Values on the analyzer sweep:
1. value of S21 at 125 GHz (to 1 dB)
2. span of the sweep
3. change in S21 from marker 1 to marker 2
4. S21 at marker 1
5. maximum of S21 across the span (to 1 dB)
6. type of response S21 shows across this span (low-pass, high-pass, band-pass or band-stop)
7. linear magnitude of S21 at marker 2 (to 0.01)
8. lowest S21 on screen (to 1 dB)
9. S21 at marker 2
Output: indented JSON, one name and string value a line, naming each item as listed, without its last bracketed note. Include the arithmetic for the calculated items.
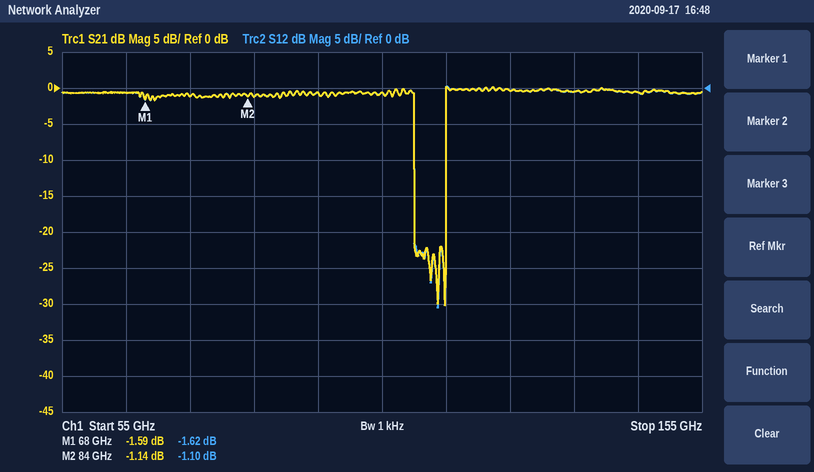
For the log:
{
  "value of S21 at 125 GHz": "0 dB",
  "span of the sweep": "100 GHz",
  "change in S21 from marker 1 to marker 2": "-1.14 − (-1.59) = 0.45 dB",
  "S21 at marker 1": "-1.59 dB",
  "maximum of S21 across the span": "0 dB",
  "type of response S21 shows across this span": "band-stop",
  "linear magnitude of S21 at marker 2": "10^(-1.14/20) ≈ 0.88",
  "lowest S21 on screen": "-30 dB",
  "S21 at marker 2": "-1.14 dB"
}
